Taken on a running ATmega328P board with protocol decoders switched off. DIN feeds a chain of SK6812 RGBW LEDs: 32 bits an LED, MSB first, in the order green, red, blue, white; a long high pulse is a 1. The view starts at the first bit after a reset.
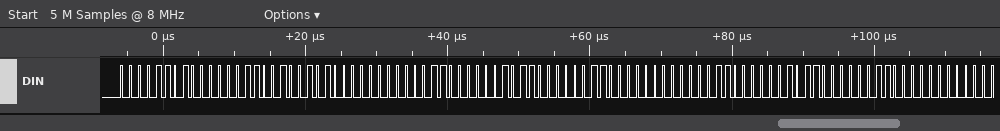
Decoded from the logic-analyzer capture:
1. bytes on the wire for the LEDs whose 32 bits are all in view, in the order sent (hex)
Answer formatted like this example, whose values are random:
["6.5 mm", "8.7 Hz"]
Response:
["0D 03 25 00 18 16 06 00 18 16 06 00"]
